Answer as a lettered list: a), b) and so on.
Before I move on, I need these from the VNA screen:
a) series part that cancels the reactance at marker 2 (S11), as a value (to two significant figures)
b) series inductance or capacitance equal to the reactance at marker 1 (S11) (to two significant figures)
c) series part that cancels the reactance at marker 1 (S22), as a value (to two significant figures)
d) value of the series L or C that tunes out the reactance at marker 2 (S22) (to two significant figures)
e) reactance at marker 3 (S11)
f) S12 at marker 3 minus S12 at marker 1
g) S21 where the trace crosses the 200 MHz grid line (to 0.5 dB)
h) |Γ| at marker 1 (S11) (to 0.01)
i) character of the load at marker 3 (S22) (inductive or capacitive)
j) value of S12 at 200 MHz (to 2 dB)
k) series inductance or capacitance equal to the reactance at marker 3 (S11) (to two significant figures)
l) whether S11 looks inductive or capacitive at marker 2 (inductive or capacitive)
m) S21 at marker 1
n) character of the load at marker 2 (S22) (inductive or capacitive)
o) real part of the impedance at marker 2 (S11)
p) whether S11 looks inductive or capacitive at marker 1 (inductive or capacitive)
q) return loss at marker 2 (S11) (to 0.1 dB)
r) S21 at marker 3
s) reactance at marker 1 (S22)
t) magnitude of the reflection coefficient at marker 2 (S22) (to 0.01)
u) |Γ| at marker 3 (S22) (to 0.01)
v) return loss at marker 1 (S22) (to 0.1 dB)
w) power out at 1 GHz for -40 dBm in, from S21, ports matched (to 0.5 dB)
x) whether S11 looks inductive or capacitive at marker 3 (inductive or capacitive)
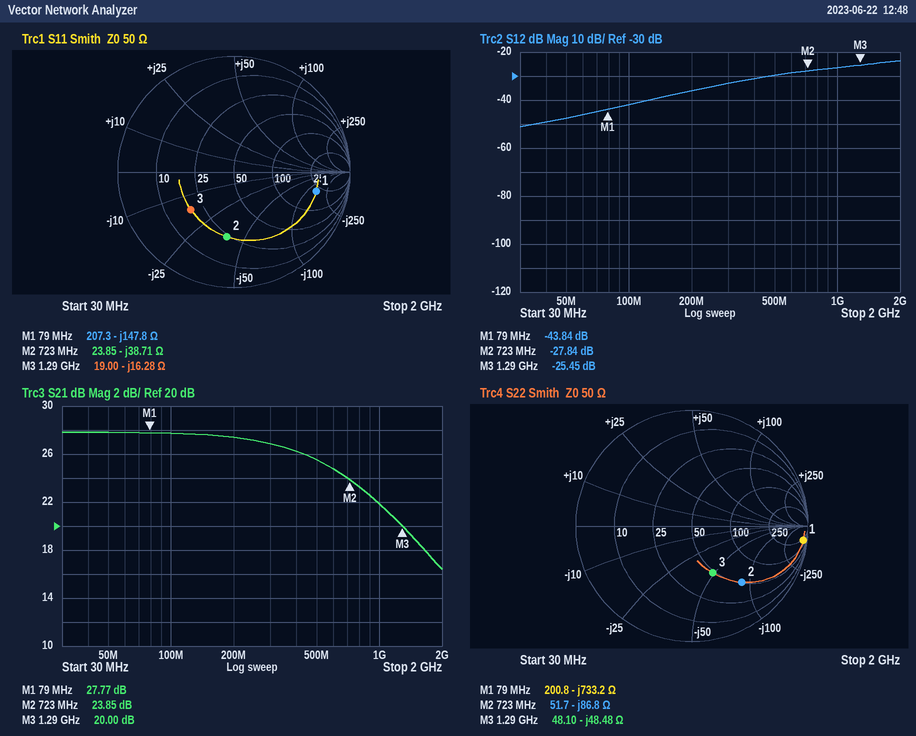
a) 8.5 nH
b) 14 pF
c) 1.5 µH
d) 19 nH
e) -16.28 Ω
f) 18.39 dB
g) 27.5 dB
h) 0.73
i) capacitive
j) -36 dB
k) 7.6 pF
l) capacitive
m) 27.77 dB
n) capacitive
o) 23.85 Ω
p) capacitive
q) 5.0 dB
r) 20.00 dB
s) -733.2 Ω
t) 0.65
u) 0.44
v) 0.3 dB
w) -18.0 dBm
x) capacitive
